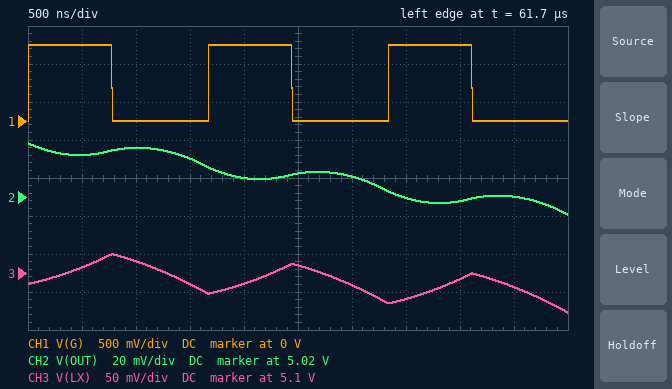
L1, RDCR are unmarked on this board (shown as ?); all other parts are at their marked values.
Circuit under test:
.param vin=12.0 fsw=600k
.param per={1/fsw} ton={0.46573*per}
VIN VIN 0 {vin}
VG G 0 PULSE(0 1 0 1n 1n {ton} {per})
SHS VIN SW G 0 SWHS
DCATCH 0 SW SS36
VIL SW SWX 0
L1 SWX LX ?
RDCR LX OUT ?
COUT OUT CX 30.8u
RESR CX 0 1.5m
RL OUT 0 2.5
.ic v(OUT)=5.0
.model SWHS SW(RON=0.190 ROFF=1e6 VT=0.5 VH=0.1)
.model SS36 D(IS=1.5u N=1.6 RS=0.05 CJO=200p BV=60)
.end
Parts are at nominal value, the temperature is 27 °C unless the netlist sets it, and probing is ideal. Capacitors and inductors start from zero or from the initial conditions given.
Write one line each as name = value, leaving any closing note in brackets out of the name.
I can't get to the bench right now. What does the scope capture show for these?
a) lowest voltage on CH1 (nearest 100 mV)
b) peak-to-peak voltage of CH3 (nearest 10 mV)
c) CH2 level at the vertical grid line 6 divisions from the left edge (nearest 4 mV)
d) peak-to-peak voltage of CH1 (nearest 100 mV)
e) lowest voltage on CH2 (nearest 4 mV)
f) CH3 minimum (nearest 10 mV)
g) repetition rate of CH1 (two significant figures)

lowest voltage on CH1 = 0 V
peak-to-peak voltage of CH3 = 80 mV
CH2 level at the vertical grid line 6 divisions from the left edge = 5.032 V
peak-to-peak voltage of CH1 = 1.0 V
lowest voltage on CH2 = 5.012 V
CH3 minimum = 5.05 V
repetition rate of CH1 = 600 kHz
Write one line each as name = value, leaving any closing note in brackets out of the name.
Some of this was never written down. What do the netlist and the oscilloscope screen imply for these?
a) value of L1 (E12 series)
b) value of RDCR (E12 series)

value of L1 = 3.9 µH
value of RDCR = 0.033 Ω
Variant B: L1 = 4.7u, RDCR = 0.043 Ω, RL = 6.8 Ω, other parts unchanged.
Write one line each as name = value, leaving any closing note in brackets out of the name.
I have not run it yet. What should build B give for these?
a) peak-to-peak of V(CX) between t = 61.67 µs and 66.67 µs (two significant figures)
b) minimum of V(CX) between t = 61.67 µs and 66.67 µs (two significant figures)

peak-to-peak of V(CX) between t = 61.67 µs and 66.67 µs = 1.7 mV
minimum of V(CX) between t = 61.67 µs and 66.67 µs = -1.0 mV
